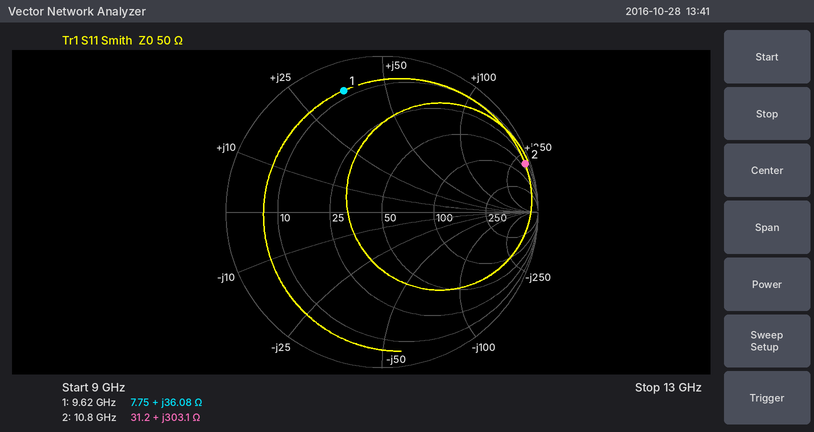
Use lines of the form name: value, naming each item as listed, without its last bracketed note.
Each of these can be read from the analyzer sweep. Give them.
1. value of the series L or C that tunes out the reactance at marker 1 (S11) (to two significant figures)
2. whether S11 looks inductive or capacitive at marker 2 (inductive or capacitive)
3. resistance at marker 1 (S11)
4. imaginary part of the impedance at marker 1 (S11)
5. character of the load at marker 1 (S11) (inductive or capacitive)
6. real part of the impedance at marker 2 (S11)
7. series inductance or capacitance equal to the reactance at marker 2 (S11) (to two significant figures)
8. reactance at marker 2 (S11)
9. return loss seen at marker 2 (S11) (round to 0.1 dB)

value of the series L or C that tunes out the reactance at marker 1 (S11): 460 fF
whether S11 looks inductive or capacitive at marker 2: inductive
resistance at marker 1: 7.75 Ω
imaginary part of the impedance at marker 1: +36.08 Ω
character of the load at marker 1 (S11): inductive
real part of the impedance at marker 2: 31.2 Ω
series inductance or capacitance equal to the reactance at marker 2 (S11): 4.5 nH
reactance at marker 2: +303.1 Ω
return loss seen at marker 2 (S11): 0.3 dB
